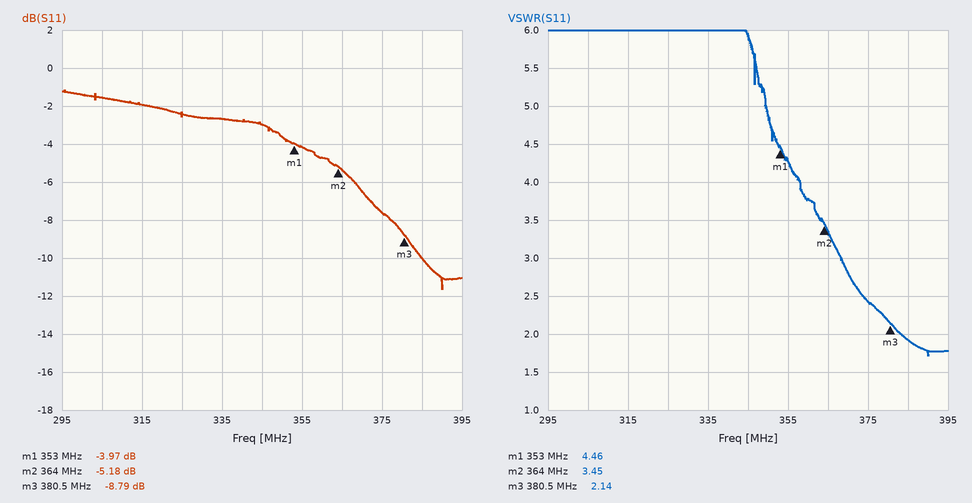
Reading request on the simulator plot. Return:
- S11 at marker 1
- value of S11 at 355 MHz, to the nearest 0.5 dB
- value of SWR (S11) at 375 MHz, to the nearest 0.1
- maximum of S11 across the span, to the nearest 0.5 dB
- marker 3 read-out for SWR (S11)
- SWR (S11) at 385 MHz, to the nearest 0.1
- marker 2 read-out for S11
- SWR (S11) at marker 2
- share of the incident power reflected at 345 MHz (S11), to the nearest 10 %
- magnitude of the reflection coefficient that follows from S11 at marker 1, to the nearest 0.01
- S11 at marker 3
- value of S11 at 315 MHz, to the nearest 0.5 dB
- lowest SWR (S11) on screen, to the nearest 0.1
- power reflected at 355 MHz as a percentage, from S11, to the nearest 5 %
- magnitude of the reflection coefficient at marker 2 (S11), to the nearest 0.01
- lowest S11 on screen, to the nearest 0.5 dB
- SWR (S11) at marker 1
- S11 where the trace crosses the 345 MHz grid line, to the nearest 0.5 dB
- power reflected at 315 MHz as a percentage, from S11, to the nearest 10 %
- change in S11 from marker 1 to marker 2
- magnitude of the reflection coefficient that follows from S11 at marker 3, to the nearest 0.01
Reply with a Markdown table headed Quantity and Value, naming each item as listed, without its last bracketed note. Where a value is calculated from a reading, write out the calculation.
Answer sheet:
| Quantity | Value |
|---|---|
| S11 at marker 1 | -3.97 dB |
| value of S11 at 355 MHz, to the nearest 0.5 dB | -4.0 dB |
| value of SWR (S11) at 375 MHz, to the nearest 0.1 | 2.4 |
| maximum of S11 across the span, to the nearest 0.5 dB | -1.0 dB |
| marker 3 read-out for SWR | 2.14 |
| SWR (S11) at 385 MHz, to the nearest 0.1 | 1.9 |
| marker 2 read-out for S11 | -5.18 dB |
| SWR (S11) at marker 2 | 3.45 |
| share of the incident power reflected at 345 MHz (S11), to the nearest 10 % | 10^(-3/10) ≈ 50 % |
| magnitude of the reflection coefficient that follows from S11 at marker 1, to the nearest 0.01 | 10^(-3.97/20) ≈ 0.63 |
| S11 at marker 3 | -8.79 dB |
| value of S11 at 315 MHz, to the nearest 0.5 dB | -2.0 dB |
| lowest SWR (S11) on screen, to the nearest 0.1 | 1.7 |
| power reflected at 355 MHz as a percentage, from S11, to the nearest 5 % | 10^(-4/10) ≈ 40 % |
| magnitude of the reflection coefficient at marker 2 (S11), to the nearest 0.01 | 10^(-5.18/20) ≈ 0.55 |
| lowest S11 on screen, to the nearest 0.5 dB | -11.5 dB |
| SWR (S11) at marker 1 | 4.46 |
| S11 where the trace crosses the 345 MHz grid line, to the nearest 0.5 dB | -3.0 dB |
| power reflected at 315 MHz as a percentage, from S11, to the nearest 10 % | 10^(-2/10) ≈ 63.1 %, so 60 % to the nearest 10 % |
| change in S11 from marker 1 to marker 2 | -5.18 − (-3.97) = -1.21 dB |
| magnitude of the reflection coefficient that follows from S11 at marker 3, to the nearest 0.01 | 10^(-8.79/20) ≈ 0.36 |
